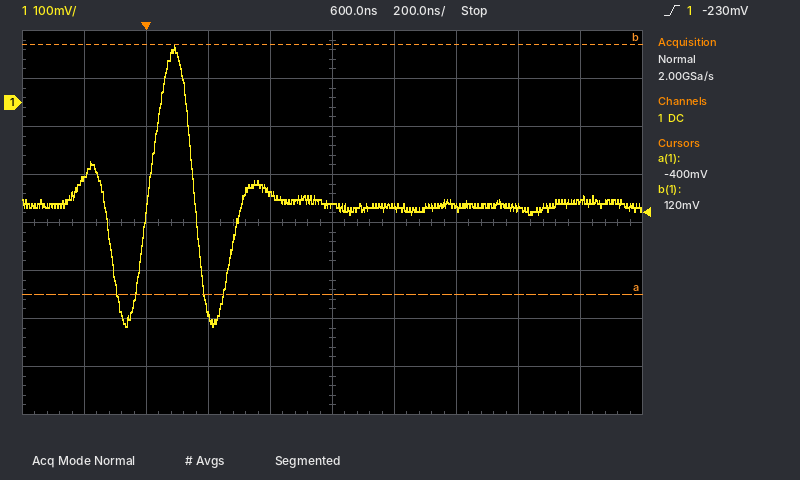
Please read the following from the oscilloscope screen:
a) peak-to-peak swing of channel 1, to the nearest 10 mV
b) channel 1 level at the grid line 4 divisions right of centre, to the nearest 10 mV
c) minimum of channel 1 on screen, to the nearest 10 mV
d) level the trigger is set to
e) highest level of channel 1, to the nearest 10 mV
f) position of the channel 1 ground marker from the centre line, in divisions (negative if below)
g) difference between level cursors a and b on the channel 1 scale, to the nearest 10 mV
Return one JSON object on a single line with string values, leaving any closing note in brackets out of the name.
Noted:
{"peak-to-peak swing of channel 1, to the nearest 10 mV": "590 mV", "channel 1 level at the grid line 4 divisions right of centre, to the nearest 10 mV": "-210 mV", "minimum of channel 1 on screen, to the nearest 10 mV": "-470 mV", "level the trigger is set to": "-230 mV", "highest level of channel 1, to the nearest 10 mV": "120 mV", "position of the channel 1 ground marker from the centre line, in divisions": "+2.5 div", "difference between level cursors a and b on the channel 1 scale, to the nearest 10 mV": "520 mV"}
